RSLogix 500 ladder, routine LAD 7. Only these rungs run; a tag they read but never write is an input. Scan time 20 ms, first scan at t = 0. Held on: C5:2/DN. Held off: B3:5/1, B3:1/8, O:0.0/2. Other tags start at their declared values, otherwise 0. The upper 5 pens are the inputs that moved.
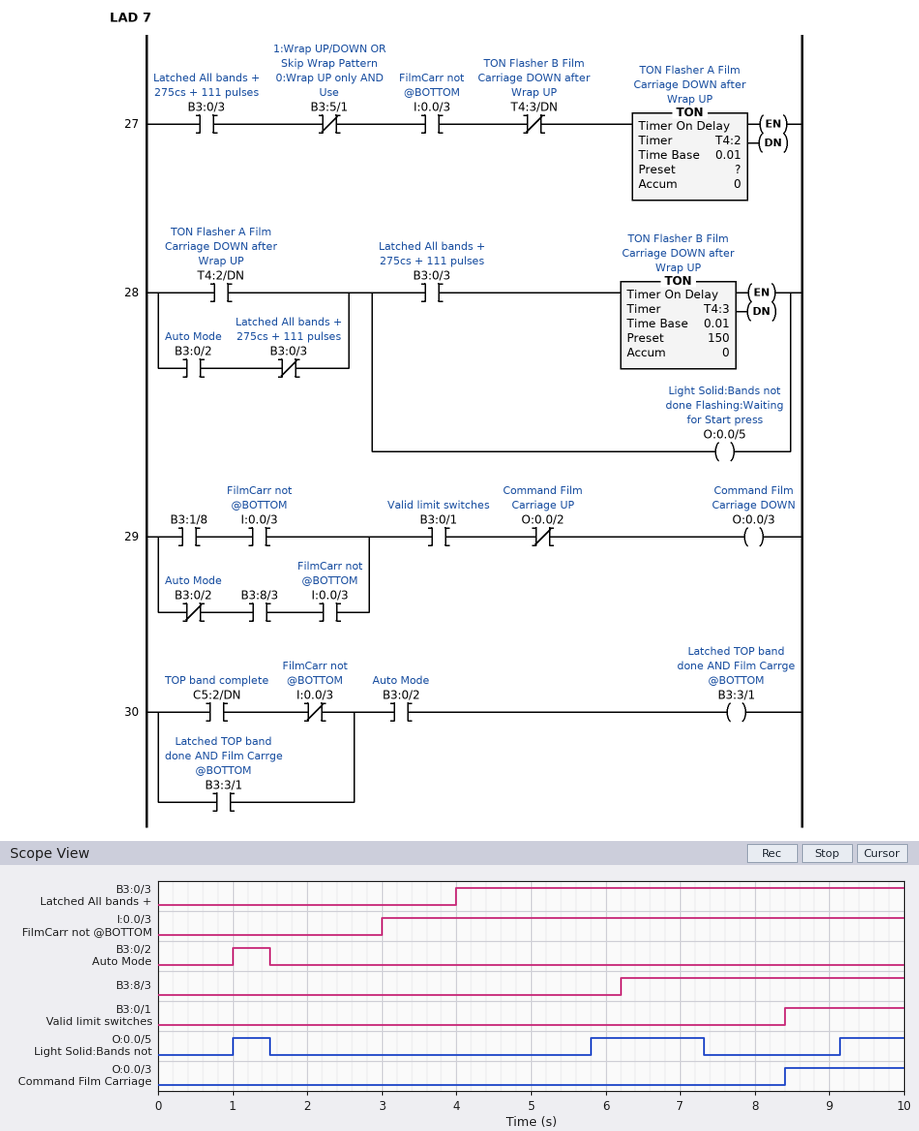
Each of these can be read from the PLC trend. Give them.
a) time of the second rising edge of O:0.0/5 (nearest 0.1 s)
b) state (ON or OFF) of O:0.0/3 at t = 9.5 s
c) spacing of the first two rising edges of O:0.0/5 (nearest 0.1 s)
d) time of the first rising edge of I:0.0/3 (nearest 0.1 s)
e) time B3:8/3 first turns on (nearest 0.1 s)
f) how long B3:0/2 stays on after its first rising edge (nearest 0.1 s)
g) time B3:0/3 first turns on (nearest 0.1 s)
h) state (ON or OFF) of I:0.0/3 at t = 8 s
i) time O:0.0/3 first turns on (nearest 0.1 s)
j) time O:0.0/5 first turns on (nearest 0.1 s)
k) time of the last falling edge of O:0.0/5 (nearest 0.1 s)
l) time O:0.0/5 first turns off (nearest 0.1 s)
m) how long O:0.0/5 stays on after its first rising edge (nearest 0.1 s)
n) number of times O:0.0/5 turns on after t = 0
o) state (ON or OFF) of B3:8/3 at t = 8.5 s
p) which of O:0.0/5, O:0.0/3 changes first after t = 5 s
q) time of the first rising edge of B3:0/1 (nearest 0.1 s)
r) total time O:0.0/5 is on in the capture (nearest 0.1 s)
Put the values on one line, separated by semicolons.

5.8 s; ON; 4.8 s; 3.0 s; 6.2 s; 0.5 s; 4.0 s; ON; 8.4 s; 1.0 s; 7.3 s; 1.5 s; 0.5 s; 3; ON; O:0.0/5; 8.4 s; 2.9 s
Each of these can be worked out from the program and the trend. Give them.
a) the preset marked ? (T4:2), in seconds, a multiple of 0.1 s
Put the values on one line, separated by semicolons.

1.8 s
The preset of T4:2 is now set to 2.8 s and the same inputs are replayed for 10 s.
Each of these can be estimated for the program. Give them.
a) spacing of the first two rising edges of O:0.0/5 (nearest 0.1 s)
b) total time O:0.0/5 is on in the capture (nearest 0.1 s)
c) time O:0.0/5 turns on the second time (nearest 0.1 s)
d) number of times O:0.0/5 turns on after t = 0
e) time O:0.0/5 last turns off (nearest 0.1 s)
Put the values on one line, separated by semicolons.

5.8 s; 2.0 s; 6.8 s; 2; 8.3 s
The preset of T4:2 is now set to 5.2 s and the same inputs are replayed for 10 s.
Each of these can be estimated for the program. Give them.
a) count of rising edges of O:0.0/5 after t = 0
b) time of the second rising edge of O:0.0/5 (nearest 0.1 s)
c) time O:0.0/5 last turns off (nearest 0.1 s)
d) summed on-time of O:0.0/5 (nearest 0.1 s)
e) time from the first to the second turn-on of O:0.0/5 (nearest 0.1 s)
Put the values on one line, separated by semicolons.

2; 9.2 s; 1.5 s; 1.3 s; 8.2 s
